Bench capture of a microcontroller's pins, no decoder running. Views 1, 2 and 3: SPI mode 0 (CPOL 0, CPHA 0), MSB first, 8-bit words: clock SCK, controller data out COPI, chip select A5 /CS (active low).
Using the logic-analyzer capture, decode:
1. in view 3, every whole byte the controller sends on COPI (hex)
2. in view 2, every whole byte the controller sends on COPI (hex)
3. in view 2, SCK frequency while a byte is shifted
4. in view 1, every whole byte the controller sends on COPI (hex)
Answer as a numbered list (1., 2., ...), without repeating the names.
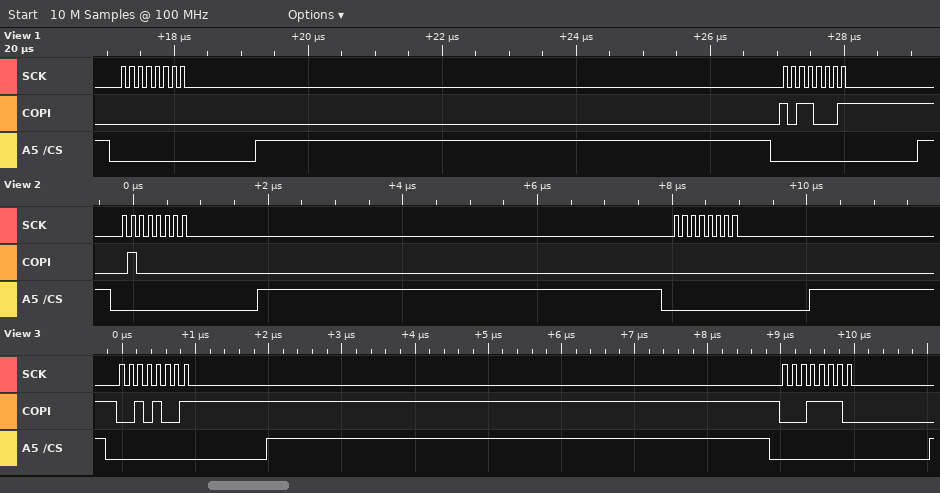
1. 29 1E
2. 0x40 0x00
3. 8 MHz
4. 0x00 0xB1
